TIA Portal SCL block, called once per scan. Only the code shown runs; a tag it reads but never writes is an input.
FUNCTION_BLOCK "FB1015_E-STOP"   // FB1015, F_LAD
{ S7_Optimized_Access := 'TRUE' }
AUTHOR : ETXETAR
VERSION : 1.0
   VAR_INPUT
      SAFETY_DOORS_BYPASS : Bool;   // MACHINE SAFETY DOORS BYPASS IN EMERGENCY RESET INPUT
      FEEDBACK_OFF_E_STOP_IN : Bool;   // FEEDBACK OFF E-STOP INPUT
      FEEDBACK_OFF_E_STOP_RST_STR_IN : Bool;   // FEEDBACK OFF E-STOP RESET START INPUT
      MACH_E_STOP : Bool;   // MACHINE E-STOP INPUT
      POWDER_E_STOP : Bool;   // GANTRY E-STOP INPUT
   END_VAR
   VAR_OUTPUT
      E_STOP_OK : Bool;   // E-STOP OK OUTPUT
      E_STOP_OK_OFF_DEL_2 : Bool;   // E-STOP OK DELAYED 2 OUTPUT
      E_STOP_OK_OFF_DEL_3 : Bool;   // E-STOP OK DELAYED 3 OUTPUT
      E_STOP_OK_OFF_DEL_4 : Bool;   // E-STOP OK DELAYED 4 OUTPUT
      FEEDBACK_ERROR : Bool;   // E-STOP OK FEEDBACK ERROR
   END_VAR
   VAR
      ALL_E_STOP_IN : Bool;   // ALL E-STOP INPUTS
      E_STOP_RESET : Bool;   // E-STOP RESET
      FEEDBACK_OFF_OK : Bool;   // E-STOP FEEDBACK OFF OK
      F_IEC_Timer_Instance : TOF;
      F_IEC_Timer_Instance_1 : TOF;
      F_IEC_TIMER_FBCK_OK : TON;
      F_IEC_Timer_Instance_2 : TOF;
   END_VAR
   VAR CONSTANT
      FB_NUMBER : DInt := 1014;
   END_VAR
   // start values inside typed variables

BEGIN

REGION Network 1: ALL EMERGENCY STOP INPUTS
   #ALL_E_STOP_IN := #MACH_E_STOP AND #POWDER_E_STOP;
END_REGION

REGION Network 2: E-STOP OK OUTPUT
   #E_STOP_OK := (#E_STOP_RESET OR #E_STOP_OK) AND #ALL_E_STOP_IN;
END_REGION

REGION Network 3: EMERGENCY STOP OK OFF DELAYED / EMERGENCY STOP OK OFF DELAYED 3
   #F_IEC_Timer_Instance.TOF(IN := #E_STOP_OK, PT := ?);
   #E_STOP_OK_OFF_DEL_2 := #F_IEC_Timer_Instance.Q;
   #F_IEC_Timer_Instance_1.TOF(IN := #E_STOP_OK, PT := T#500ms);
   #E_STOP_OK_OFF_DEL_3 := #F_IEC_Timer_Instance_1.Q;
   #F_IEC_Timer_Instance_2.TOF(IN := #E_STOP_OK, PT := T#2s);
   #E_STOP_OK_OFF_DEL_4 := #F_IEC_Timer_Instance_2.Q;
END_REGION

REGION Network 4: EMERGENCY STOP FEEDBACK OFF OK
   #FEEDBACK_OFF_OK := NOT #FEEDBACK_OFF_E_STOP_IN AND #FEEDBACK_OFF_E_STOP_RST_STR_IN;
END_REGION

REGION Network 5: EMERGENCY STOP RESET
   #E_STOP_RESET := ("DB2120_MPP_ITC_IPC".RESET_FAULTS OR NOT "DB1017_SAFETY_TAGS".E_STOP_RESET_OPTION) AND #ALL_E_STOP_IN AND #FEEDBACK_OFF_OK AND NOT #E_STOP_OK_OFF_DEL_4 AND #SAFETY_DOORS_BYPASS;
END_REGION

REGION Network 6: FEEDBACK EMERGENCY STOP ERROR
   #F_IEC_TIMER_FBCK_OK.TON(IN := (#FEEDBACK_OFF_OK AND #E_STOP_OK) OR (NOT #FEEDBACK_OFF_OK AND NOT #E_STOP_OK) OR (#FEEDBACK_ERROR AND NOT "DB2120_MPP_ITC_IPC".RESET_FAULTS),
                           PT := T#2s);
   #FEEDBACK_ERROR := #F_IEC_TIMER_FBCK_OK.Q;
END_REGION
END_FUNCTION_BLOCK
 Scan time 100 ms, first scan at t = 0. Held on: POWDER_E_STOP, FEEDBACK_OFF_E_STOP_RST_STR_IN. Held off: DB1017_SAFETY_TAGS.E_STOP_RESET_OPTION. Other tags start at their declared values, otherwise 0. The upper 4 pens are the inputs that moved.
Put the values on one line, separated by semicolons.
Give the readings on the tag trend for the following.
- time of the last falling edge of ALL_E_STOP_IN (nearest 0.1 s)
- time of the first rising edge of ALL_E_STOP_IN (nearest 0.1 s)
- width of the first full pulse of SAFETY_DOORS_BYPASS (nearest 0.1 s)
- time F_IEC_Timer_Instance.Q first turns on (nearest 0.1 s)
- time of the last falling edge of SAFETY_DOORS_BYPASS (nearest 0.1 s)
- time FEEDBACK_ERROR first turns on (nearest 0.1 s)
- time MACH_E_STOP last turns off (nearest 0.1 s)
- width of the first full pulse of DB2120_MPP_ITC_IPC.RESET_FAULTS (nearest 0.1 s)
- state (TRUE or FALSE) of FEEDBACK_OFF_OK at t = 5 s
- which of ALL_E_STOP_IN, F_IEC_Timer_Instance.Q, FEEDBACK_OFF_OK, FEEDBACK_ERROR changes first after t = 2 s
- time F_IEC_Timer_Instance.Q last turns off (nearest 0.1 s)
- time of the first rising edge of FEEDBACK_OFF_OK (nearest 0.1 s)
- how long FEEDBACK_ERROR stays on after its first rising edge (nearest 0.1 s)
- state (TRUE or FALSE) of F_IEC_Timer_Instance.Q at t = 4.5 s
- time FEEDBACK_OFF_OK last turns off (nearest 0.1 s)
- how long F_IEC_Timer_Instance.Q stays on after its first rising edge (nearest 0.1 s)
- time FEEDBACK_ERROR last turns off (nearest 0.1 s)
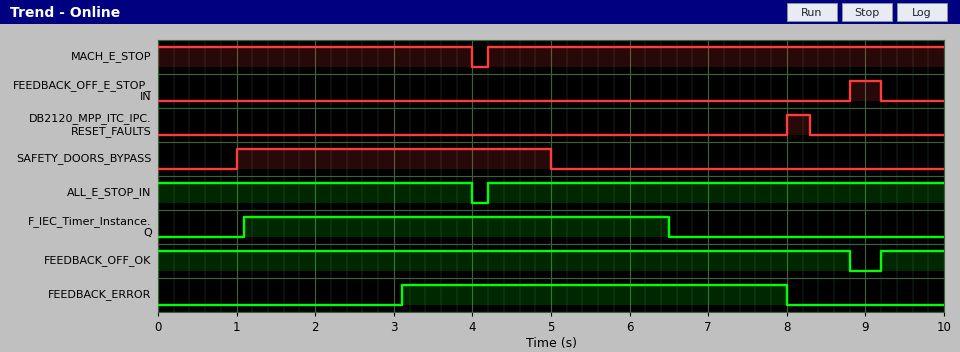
4.0 s; 4.2 s; 4.0 s; 1.1 s; 5.0 s; 3.1 s; 4.0 s; 0.3 s; TRUE; FEEDBACK_ERROR; 6.5 s; 9.2 s; 4.9 s; TRUE; 8.8 s; 5.4 s; 8.0 s
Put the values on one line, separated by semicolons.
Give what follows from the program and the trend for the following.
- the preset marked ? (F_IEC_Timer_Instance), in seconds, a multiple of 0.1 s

2.5 s
